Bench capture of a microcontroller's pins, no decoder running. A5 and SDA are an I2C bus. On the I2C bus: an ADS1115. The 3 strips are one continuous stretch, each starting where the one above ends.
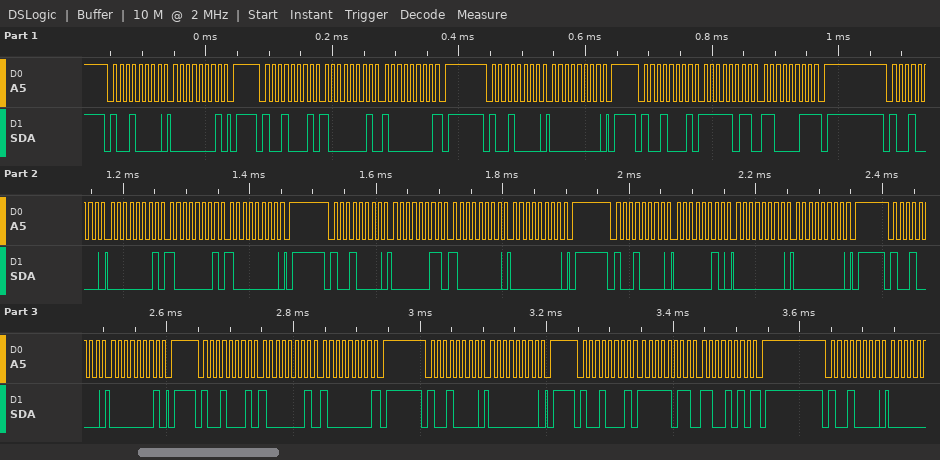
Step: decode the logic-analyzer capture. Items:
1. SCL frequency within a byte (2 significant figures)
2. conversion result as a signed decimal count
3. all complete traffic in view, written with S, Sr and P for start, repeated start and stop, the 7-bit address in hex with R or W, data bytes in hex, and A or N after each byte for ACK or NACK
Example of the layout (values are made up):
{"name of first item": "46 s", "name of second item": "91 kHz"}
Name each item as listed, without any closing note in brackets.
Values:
{"SCL frequency within a byte": "100 kHz", "conversion result as a signed decimal count": "-1085", "all complete traffic in view, written with S, Sr and P for start, repeated start and stop, the 7-bit address in hex with R or W, data bytes in hex, and A or N after each byte for ACK or NACK": "S 48W A 01 A P S 48R A 81 A 80 N P S 48W A 00 A P S 48R A FB A C3 N P S 48W A 01 A 81 A 80 A P S 48W A 03 A 80 A 00 A P S 48W A 02 A 00 A 00 A P S 48W A 01 A P S 48R A 81 A 80 N P S 48W A 00 A P S 48R A FB A CA N P S 48W A"}
